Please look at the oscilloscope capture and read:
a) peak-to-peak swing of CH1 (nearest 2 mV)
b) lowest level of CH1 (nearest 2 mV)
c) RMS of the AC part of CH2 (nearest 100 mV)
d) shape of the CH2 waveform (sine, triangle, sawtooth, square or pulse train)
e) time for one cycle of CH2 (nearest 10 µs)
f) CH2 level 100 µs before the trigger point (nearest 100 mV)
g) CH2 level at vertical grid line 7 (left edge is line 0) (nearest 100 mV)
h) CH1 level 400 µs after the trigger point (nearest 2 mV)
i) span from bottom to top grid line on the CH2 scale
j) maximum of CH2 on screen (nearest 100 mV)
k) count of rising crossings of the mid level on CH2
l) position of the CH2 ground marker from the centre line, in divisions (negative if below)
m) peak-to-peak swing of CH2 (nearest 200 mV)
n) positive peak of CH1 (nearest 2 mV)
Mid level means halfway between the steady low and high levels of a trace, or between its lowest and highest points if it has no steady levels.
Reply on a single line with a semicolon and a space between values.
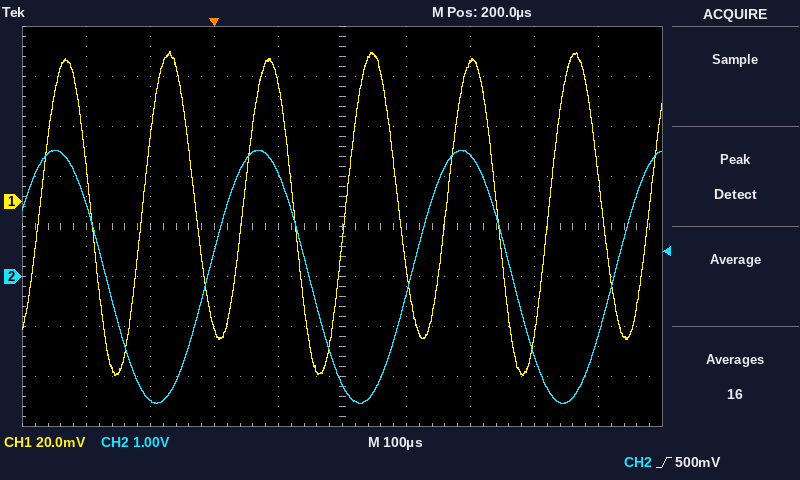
130 mV; -70 mV; 1.8 V; sine; 320 µs; -2.5 V; 2.4 V; 56 mV; 8 V; 2.5 V; 3; -1.0 div; 5.0 V; 60 mV
